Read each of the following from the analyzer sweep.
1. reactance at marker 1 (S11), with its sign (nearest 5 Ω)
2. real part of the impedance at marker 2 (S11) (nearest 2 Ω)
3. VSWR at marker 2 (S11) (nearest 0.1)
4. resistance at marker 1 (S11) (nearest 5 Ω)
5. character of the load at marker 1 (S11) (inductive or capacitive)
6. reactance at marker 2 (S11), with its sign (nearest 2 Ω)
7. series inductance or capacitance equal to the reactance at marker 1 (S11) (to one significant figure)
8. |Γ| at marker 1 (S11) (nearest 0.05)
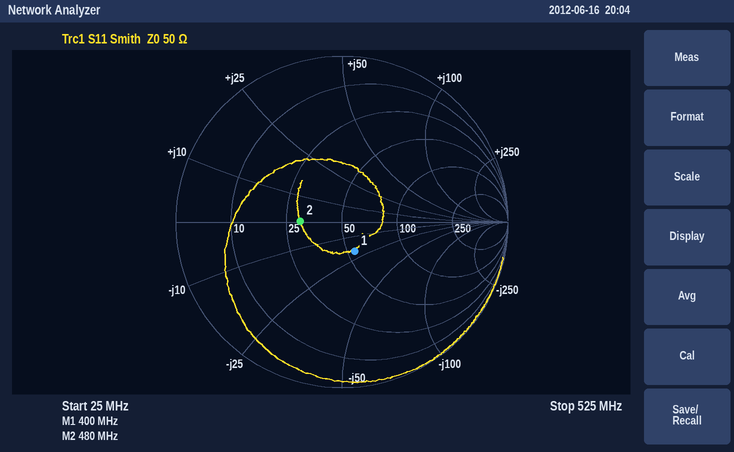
-20 Ω
30 Ω
1.7
55 Ω
capacitive
0 Ω
20 pF
0.20
